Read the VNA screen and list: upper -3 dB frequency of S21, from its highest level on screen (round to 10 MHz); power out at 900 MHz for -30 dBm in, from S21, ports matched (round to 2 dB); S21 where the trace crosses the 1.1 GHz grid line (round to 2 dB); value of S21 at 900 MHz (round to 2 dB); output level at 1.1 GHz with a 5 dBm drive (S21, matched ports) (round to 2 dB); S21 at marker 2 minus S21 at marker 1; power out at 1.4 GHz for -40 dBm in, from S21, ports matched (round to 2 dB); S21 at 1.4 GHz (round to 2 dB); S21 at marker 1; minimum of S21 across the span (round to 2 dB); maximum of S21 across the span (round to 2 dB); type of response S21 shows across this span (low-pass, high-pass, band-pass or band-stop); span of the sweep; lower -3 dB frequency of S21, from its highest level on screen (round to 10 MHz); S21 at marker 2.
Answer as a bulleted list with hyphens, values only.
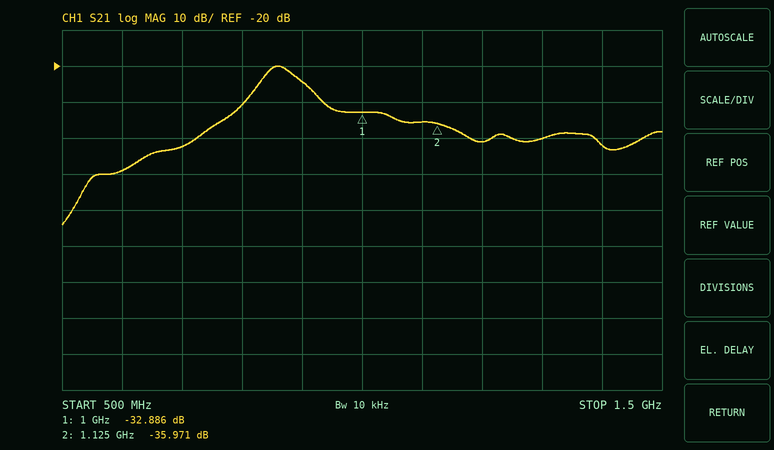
- 890 MHz
- -54 dBm
- -36 dB
- -24 dB
- -30 dBm
- -3.085 dB
- -82 dBm
- -42 dB
- -32.886 dB
- -64 dB
- -20 dB
- band-pass
- 1 GHz
- 840 MHz
- -35.971 dB
